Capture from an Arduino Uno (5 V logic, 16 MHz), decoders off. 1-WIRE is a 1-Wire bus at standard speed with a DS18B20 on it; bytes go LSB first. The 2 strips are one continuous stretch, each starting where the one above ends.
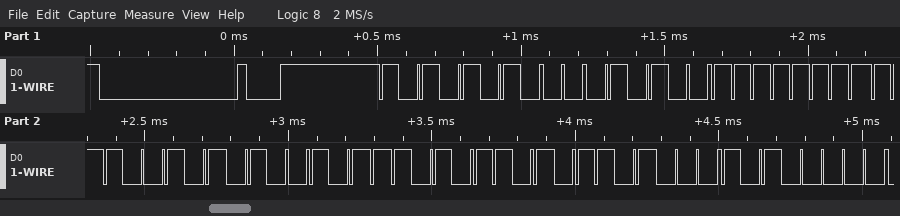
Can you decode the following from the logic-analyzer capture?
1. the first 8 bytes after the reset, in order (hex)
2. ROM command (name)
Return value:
55 28 FF A7 D2 B5 16 05
Match ROM
